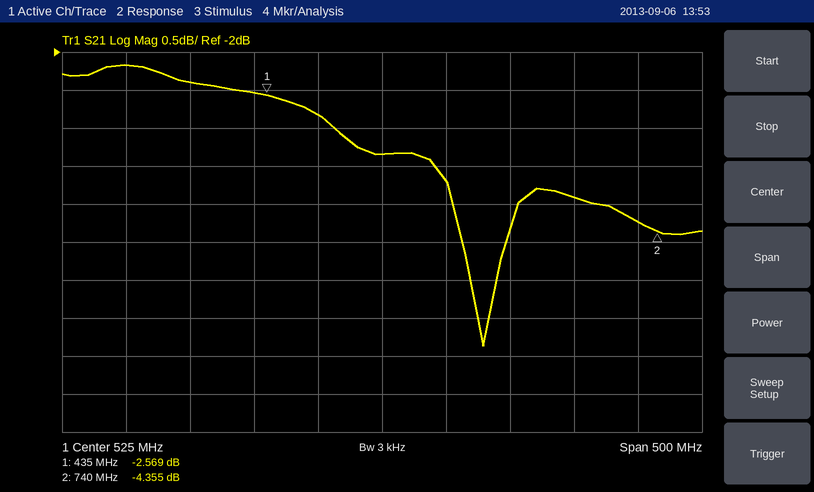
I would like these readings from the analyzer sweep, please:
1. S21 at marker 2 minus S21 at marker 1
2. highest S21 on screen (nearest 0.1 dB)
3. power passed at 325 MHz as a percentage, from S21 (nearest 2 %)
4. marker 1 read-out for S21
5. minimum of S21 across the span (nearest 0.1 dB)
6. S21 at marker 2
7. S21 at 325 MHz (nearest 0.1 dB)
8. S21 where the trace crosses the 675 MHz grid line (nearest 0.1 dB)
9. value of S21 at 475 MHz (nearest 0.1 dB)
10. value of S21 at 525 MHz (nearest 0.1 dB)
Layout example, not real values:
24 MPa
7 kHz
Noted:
-1.786 dB
-2.2 dB
60 %
-2.569 dB
-5.9 dB
-4.355 dB
-2.2 dB
-3.9 dB
-2.8 dB
-3.3 dB
